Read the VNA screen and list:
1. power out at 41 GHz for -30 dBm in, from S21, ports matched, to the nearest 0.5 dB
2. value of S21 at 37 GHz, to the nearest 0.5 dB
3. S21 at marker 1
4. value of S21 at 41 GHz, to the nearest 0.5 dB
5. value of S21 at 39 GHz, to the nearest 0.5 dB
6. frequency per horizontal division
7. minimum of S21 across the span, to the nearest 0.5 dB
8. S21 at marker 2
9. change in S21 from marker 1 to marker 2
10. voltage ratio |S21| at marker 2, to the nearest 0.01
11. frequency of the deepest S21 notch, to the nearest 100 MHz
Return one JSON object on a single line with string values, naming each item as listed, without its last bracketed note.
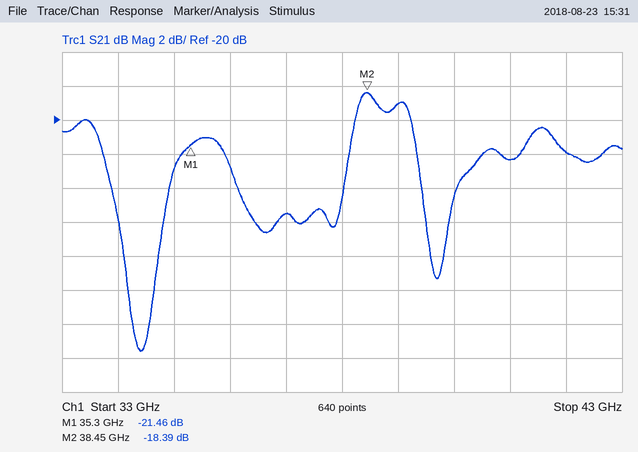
{"power out at 41 GHz for -30 dBm in, from S21, ports matched, to the nearest 0.5 dB": "-52.5 dBm", "value of S21 at 37 GHz, to the nearest 0.5 dB": "-25.5 dB", "S21 at marker 1": "-21.46 dB", "value of S21 at 41 GHz, to the nearest 0.5 dB": "-22.5 dB", "value of S21 at 39 GHz, to the nearest 0.5 dB": "-19.0 dB", "frequency per horizontal division": "1 GHz", "minimum of S21 across the span, to the nearest 0.5 dB": "-33.5 dB", "S21 at marker 2": "-18.39 dB", "change in S21 from marker 1 to marker 2": "3.07 dB", "voltage ratio |S21| at marker 2, to the nearest 0.01": "0.12", "frequency of the deepest S21 notch, to the nearest 100 MHz": "34.4 GHz"}
